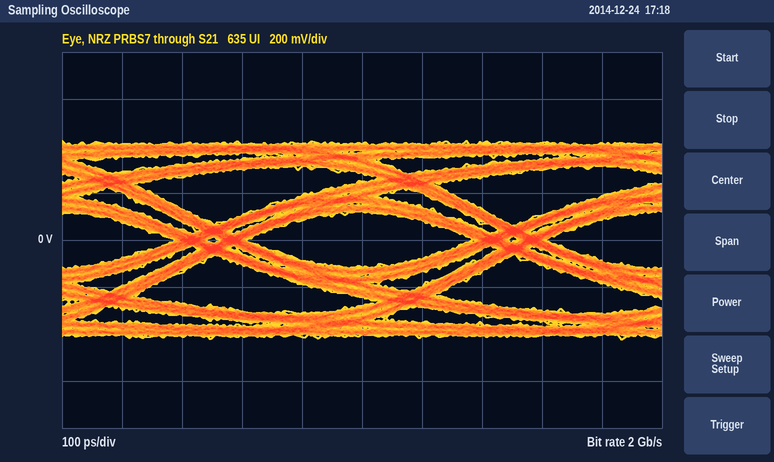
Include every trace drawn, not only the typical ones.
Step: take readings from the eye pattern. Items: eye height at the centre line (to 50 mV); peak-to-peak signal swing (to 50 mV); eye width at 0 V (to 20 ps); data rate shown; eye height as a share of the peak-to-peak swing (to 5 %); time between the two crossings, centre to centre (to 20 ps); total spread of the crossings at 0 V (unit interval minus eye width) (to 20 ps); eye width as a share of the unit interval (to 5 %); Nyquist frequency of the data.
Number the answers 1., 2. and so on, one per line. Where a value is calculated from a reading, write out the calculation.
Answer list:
1. 250 mV
2. 850 mV
3. 380 ps
4. 2 Gb/s
5. 250 mV / 850 mV ≈ 29.4 %, so 30 % to the nearest 5 %
6. 500 ps
7. 120 ps
8. 380 ps / 500 ps ≈ 76.0 %, so 75 % to the nearest 5 %
9. 1 GHz
